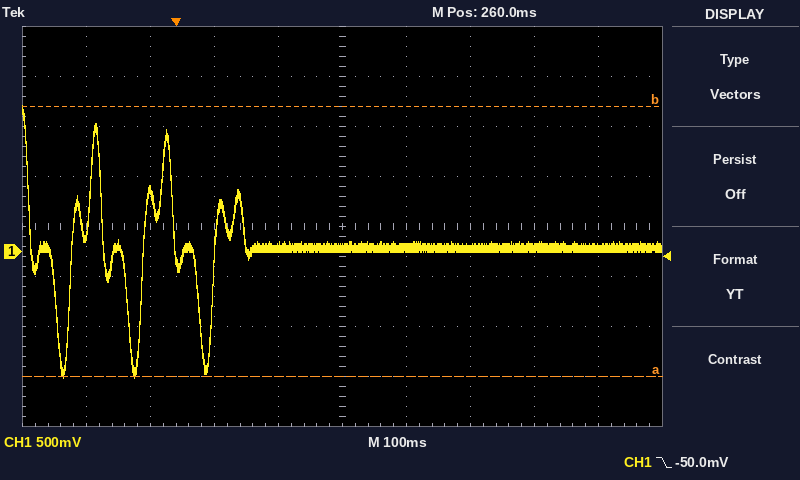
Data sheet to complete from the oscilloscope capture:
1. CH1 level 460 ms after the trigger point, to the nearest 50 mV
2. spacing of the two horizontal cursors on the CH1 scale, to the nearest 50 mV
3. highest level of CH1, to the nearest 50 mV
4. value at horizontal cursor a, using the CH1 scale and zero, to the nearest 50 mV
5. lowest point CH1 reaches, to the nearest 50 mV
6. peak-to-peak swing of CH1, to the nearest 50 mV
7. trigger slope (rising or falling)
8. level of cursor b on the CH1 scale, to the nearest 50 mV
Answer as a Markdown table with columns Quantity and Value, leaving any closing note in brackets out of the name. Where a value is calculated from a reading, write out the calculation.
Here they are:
| Quantity | Value |
|---|---|
| CH1 level 460 ms after the trigger point, to the nearest 50 mV | 50 mV |
| spacing of the two horizontal cursors on the CH1 scale, to the nearest 50 mV | 2.70 V |
| highest level of CH1, to the nearest 50 mV | 1.45 V |
| value at horizontal cursor a, using the CH1 scale and zero, to the nearest 50 mV | -1.25 V |
| lowest point CH1 reaches, to the nearest 50 mV | -1.25 V |
| peak-to-peak swing of CH1, to the nearest 50 mV | 1.45 V − (-1.25 V) = 2.70 V |
| trigger slope | falling |
| level of cursor b on the CH1 scale, to the nearest 50 mV | 1.45 V |
